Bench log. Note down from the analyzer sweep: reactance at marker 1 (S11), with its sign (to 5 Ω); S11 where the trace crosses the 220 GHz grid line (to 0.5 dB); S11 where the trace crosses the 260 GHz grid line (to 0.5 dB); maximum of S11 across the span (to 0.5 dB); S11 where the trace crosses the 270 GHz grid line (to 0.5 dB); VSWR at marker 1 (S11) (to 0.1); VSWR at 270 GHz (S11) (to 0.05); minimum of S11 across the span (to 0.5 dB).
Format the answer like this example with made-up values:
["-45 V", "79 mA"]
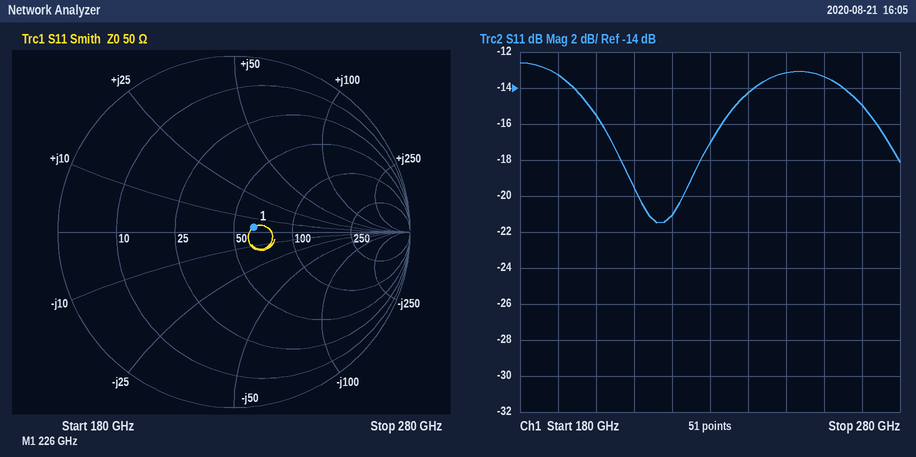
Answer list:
["+5 Ω", "-21.0 dB", "-13.5 dB", "-12.5 dB", "-15.0 dB", "1.3", "1.45", "-21.5 dB"]
